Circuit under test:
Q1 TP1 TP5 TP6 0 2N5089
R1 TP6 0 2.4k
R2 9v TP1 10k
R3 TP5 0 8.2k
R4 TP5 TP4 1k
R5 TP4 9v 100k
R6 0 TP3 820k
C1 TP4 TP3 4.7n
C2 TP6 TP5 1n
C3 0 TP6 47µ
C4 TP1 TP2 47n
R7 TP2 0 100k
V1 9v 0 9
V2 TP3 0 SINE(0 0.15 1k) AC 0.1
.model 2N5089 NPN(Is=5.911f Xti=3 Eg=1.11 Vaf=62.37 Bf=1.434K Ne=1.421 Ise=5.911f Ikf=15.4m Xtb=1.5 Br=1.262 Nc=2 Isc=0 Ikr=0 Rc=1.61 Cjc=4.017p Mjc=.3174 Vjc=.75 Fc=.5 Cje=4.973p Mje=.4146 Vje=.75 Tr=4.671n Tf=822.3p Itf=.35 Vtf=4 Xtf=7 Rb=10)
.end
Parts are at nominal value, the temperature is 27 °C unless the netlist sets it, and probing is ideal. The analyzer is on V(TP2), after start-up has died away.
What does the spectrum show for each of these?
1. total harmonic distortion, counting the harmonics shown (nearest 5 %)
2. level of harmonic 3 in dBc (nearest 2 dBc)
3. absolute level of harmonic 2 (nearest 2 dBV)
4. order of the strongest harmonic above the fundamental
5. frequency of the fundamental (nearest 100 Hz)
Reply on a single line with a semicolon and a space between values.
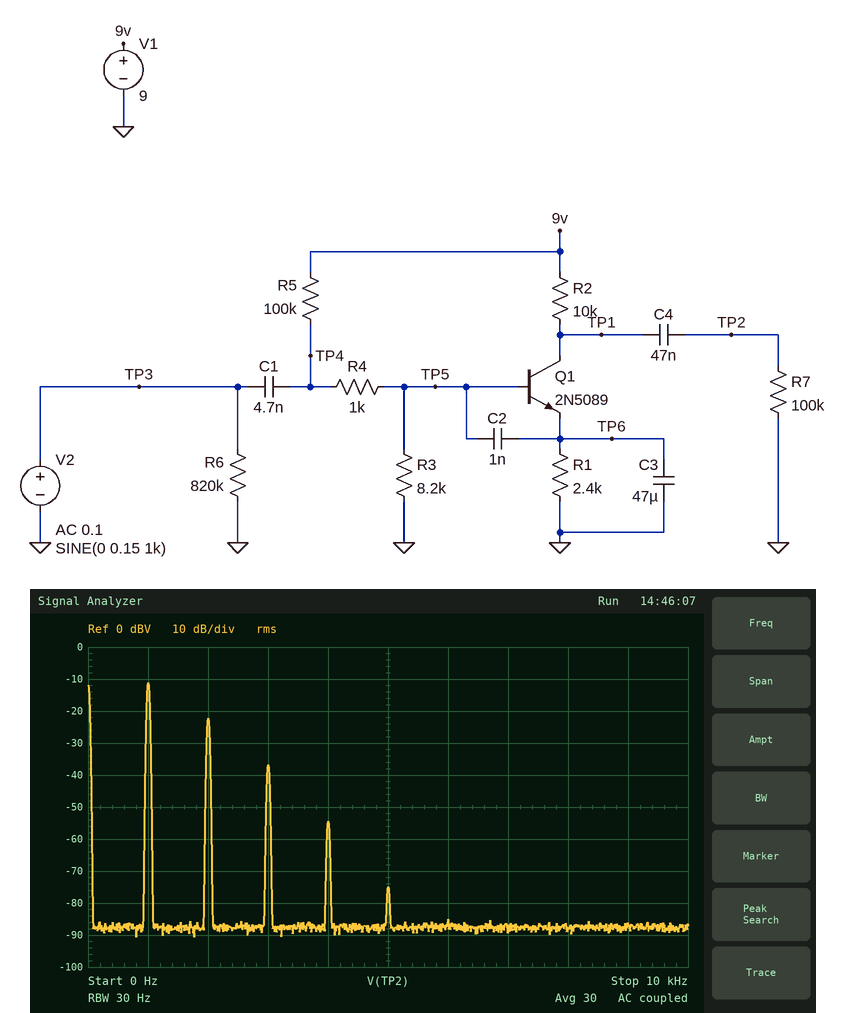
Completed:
30 %; -26 dBc; -22 dBV; 2; 1.0 kHz
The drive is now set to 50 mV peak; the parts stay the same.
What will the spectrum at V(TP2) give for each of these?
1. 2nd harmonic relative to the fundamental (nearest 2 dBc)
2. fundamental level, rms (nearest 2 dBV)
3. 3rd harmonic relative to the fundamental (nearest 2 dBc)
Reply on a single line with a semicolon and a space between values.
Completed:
-20 dBc; -20 dBV; -44 dBc
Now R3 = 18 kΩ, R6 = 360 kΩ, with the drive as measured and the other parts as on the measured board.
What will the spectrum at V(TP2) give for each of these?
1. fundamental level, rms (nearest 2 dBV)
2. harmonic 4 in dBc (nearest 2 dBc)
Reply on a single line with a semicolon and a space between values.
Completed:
8 dBV; -36 dBc
